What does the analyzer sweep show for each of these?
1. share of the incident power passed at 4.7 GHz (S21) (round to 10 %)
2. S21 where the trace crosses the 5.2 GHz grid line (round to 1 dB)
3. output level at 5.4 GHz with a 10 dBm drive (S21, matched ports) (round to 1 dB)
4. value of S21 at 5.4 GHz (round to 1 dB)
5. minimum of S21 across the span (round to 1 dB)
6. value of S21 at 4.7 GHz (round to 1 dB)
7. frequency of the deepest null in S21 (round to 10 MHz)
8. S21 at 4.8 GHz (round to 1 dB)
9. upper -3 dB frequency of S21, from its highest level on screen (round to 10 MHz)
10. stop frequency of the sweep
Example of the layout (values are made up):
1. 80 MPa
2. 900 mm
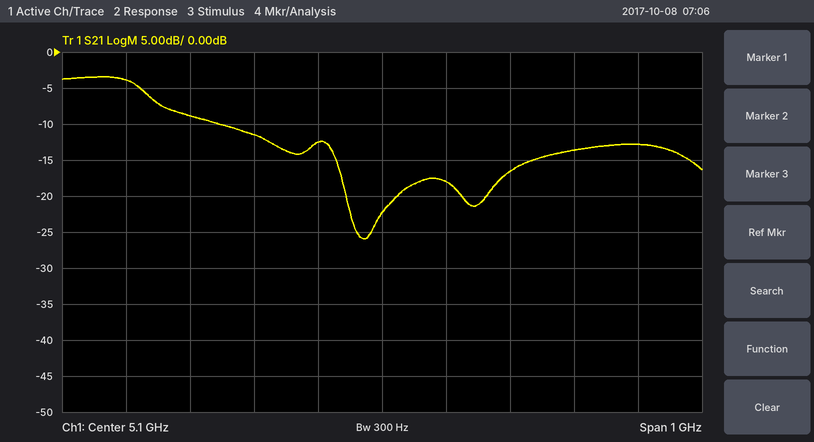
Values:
1. 40 %
2. -18 dB
3. -4 dBm
4. -14 dB
5. -26 dB
6. -4 dB
7. 5.07 GHz
8. -9 dB
9. 4.74 GHz
10. 5.6 GHz
